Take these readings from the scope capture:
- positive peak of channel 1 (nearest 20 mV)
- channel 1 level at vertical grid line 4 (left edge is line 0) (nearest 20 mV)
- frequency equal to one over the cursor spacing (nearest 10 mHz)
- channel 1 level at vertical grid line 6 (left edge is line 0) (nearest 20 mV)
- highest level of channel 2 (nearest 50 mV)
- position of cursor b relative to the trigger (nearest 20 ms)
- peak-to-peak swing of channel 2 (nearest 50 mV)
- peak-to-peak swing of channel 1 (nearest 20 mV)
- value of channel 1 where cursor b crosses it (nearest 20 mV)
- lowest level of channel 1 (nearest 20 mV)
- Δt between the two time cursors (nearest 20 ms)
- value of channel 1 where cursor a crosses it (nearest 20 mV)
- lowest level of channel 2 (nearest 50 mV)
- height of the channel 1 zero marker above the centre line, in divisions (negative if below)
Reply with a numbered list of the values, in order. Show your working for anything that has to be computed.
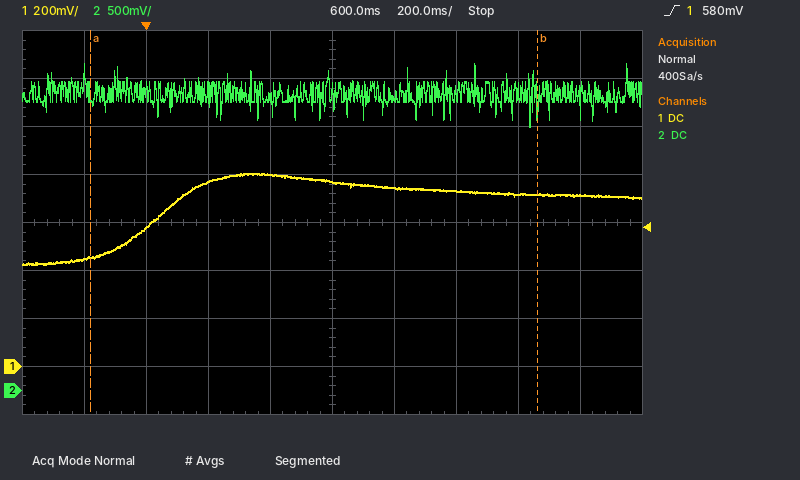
1. 800 mV
2. 800 mV
3. 1 / 1.44 s ≈ 690 mHz
4. 740 mV
5. 3.40 V
6. +1.26 s
7. 3.40 V − (2.75 V) = 650 mV
8. 800 mV − (420 mV) = 380 mV
9. 720 mV
10. 420 mV
11. 1.44 s
12. 460 mV
13. 2.75 V
14. -3.0 div
